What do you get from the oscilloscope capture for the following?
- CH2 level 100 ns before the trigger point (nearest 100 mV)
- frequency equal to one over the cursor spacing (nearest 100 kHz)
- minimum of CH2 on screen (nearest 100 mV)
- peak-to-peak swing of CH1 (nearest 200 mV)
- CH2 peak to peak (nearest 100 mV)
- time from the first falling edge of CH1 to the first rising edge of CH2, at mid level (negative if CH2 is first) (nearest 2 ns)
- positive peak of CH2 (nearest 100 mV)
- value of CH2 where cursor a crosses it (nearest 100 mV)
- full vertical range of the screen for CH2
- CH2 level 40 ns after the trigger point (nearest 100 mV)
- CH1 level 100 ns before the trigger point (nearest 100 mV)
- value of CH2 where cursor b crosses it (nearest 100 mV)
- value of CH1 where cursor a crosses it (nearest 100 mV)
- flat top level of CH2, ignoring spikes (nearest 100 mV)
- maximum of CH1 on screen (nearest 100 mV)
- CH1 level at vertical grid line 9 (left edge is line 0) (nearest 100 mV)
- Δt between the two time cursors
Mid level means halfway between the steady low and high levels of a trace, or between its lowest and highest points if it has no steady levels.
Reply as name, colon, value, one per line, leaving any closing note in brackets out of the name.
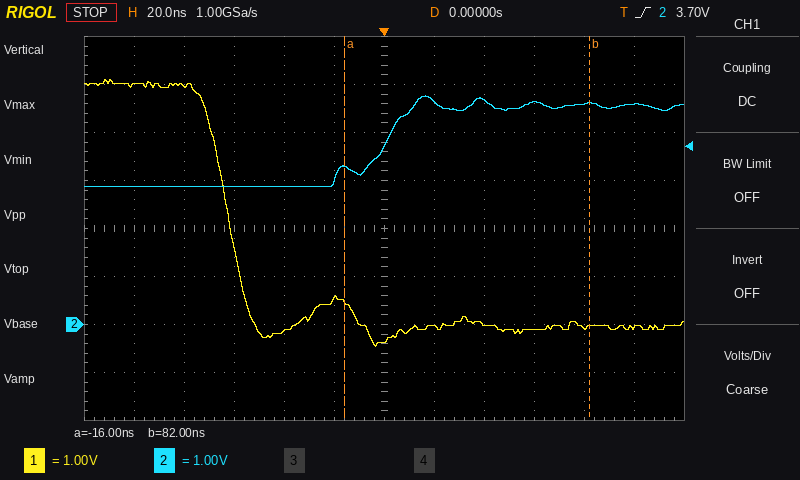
CH2 level 100 ns before the trigger point: 2.9 V
frequency equal to one over the cursor spacing: 10.2 MHz
minimum of CH2 on screen: 2.9 V
peak-to-peak swing of CH1: 5.6 V
CH2 peak to peak: 1.9 V
time from the first falling edge of CH1 to the first rising edge of CH2, at mid level (negative if CH2 is first): +62 ns
positive peak of CH2: 4.8 V
value of CH2 where cursor a crosses it: 3.3 V
full vertical range of the screen for CH2: 8 V
CH2 level 40 ns after the trigger point: 4.7 V
CH1 level 100 ns before the trigger point: 5.0 V
value of CH2 where cursor b crosses it: 4.6 V
value of CH1 where cursor a crosses it: 500 mV
flat top level of CH2, ignoring spikes: 4.5 V
maximum of CH1 on screen: 5.1 V
CH1 level at vertical grid line 9 (left edge is line 0): -100 mV
Δt between the two time cursors: 98 ns
